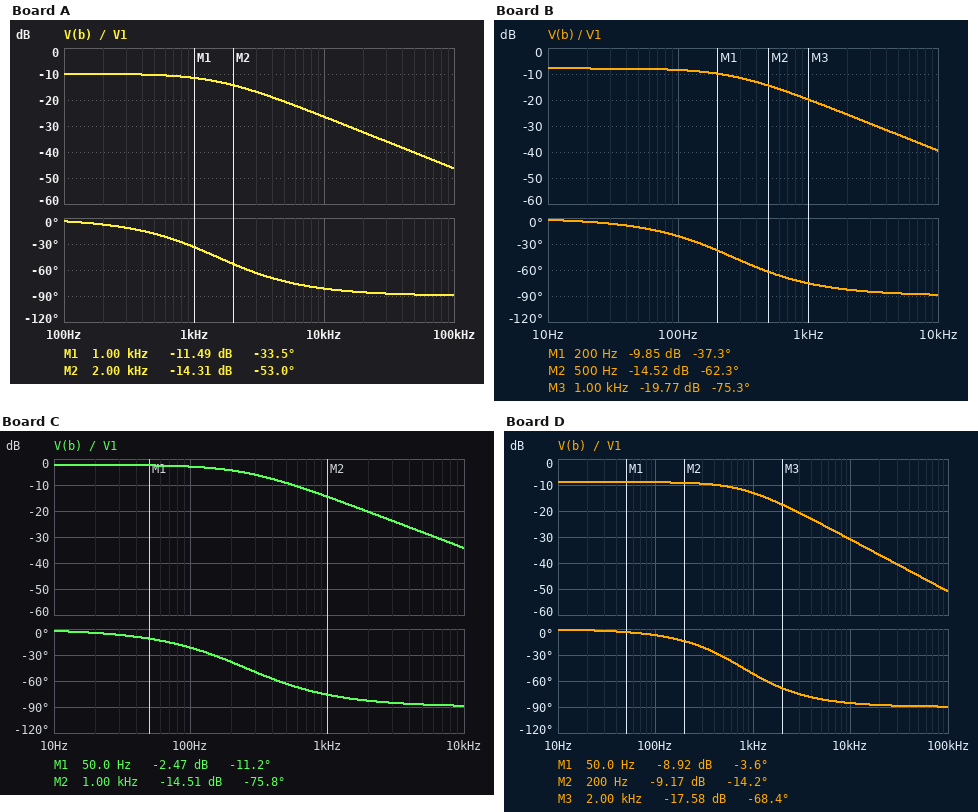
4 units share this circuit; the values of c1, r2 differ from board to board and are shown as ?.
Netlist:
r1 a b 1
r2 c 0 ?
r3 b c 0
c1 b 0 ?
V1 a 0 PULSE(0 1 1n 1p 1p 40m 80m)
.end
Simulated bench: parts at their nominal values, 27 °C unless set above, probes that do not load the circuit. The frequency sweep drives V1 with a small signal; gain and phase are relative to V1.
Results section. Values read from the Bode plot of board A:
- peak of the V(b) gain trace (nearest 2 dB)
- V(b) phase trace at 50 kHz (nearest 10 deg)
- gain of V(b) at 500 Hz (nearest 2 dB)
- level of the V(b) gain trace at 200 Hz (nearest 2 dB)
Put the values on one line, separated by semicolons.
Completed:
-10 dB; -90 deg; -10 dB; -10 dB
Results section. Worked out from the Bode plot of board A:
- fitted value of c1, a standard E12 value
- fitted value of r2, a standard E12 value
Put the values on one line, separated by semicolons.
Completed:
330 µF; 0.47 Ω
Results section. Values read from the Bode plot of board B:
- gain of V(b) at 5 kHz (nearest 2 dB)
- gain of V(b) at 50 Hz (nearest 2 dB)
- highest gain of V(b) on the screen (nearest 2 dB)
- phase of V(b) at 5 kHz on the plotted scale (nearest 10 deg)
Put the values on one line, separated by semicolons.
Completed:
-34 dB; -8 dB; -8 dB; -90 deg
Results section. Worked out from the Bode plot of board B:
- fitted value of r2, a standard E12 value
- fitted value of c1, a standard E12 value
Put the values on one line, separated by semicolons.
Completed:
0.68 Ω; 1.5 mF
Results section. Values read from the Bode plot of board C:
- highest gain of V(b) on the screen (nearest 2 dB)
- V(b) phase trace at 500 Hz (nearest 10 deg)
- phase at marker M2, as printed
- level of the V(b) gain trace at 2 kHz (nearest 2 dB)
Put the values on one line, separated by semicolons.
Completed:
-2 dB; -60 deg; -75.8 deg; -20 dB
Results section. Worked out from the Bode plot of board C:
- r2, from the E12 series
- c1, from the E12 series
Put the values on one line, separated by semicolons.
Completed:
3.3 Ω; 820 µF
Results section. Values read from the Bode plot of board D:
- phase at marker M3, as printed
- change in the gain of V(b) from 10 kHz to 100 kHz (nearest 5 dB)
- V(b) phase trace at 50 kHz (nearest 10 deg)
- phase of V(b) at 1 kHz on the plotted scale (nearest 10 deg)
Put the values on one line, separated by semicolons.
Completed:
-68.4 deg; -20 dB; -90 deg; -50 deg
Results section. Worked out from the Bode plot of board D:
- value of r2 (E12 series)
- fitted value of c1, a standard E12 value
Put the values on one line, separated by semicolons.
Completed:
0.56 Ω; 560 µF
